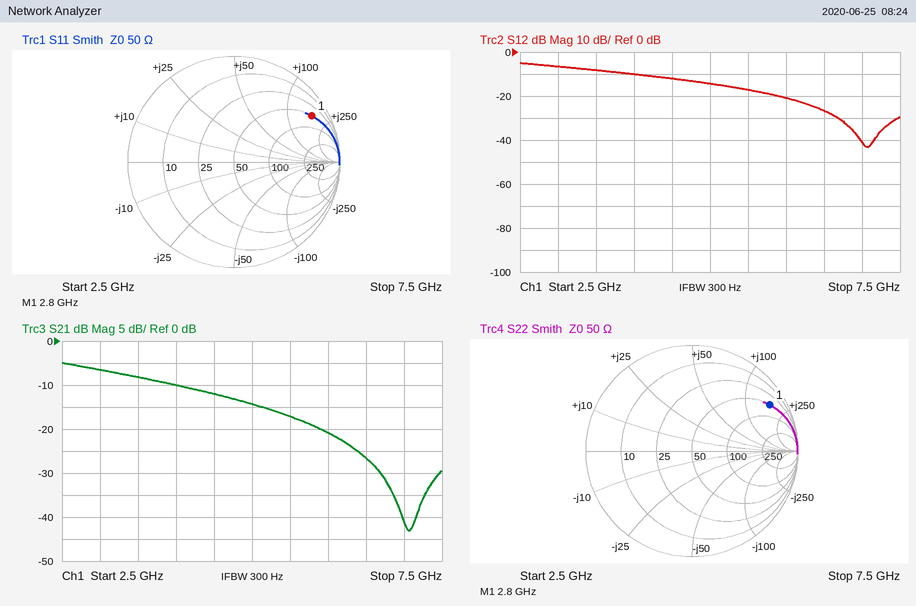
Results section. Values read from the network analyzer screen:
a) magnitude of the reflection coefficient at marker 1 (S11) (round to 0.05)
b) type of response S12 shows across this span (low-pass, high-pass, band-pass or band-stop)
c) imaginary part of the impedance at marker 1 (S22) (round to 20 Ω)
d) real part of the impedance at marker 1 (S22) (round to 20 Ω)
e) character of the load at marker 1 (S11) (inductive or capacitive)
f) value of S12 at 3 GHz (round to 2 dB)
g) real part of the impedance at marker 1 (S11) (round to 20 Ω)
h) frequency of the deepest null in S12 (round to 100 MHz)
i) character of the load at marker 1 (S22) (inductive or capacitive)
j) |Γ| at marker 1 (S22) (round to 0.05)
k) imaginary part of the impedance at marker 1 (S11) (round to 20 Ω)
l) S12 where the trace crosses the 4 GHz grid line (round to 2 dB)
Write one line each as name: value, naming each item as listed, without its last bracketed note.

magnitude of the reflection coefficient at marker 1 (S11): 0.85
type of response S12 shows across this span: low-pass
imaginary part of the impedance at marker 1 (S22): +160 Ω
real part of the impedance at marker 1 (S22): 60 Ω
character of the load at marker 1 (S11): inductive
value of S12 at 3 GHz: -6 dB
real part of the impedance at marker 1 (S11): 60 Ω
frequency of the deepest null in S12: 7.1 GHz
character of the load at marker 1 (S22): inductive
|Γ| at marker 1 (S22): 0.85
imaginary part of the impedance at marker 1 (S11): +160 Ω
S12 where the trace crosses the 4 GHz grid line: -10 dB
